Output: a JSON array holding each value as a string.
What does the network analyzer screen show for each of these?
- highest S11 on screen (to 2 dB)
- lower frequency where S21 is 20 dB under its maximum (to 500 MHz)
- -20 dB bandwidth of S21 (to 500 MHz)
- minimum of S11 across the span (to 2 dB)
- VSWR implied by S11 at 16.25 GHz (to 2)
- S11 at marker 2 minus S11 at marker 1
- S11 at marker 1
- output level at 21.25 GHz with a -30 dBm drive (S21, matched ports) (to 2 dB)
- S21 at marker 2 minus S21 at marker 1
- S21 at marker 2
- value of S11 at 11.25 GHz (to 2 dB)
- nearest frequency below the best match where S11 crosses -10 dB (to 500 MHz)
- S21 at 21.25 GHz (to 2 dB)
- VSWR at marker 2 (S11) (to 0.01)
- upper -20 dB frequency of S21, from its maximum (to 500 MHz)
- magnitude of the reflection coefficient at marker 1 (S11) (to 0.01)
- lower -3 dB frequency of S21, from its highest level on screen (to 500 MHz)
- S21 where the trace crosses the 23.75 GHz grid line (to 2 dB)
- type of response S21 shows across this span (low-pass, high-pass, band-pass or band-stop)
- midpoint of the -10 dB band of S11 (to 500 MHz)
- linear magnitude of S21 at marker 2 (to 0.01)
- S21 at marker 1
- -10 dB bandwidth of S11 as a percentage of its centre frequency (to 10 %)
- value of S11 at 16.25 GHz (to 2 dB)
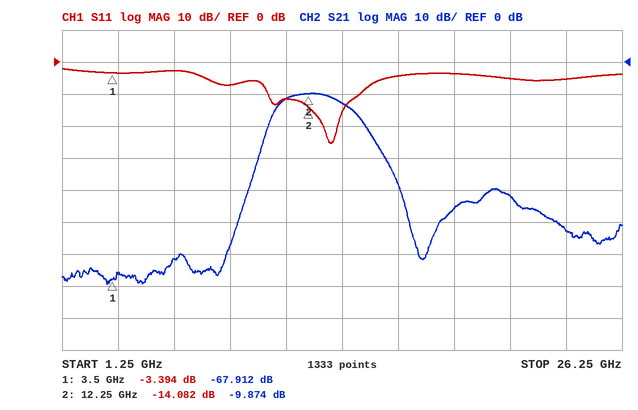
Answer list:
["-2 dB", "10.0 GHz", "5.5 GHz", "-26 dB", "4", "-10.688 dB", "-3.394 dB", "-72 dBm", "58.038 dB", "-9.874 dB", "-12 dB", "10.5 GHz", "-42 dB", "1.49", "15.5 GHz", "0.68", "11.0 GHz", "-52 dB", "band-pass", "12.5 GHz", "0.32", "-67.912 dB", "30 %", "-4 dB"]
